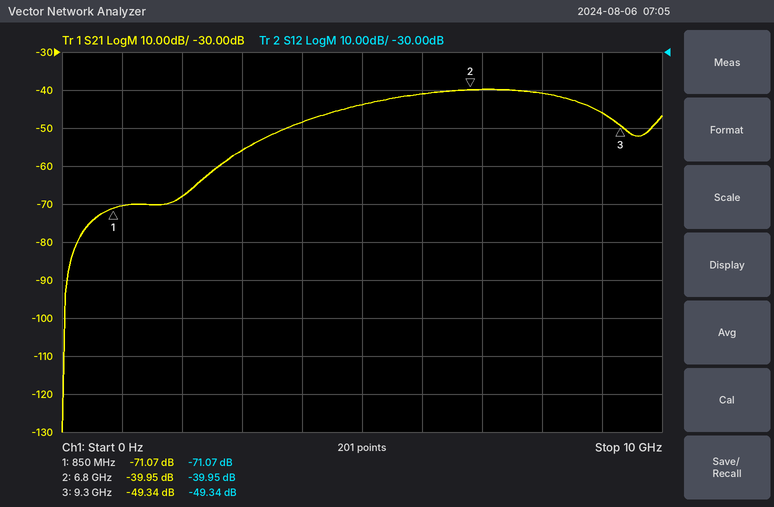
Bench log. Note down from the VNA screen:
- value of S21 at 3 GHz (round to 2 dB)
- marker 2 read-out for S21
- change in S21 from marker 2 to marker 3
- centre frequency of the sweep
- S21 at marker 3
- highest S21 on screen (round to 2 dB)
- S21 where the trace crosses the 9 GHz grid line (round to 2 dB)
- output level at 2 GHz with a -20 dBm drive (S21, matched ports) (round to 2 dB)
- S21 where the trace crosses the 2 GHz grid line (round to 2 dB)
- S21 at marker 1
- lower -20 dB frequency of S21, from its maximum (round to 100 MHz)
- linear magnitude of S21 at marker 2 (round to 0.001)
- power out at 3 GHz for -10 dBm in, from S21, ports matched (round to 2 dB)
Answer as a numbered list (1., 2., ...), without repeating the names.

1. -56 dB
2. -39.95 dB
3. -9.39 dB
4. 5 GHz
5. -49.34 dB
6. -40 dB
7. -46 dB
8. -88 dBm
9. -68 dB
10. -71.07 dB
11. 2.6 GHz
12. 0.010
13. -66 dBm
